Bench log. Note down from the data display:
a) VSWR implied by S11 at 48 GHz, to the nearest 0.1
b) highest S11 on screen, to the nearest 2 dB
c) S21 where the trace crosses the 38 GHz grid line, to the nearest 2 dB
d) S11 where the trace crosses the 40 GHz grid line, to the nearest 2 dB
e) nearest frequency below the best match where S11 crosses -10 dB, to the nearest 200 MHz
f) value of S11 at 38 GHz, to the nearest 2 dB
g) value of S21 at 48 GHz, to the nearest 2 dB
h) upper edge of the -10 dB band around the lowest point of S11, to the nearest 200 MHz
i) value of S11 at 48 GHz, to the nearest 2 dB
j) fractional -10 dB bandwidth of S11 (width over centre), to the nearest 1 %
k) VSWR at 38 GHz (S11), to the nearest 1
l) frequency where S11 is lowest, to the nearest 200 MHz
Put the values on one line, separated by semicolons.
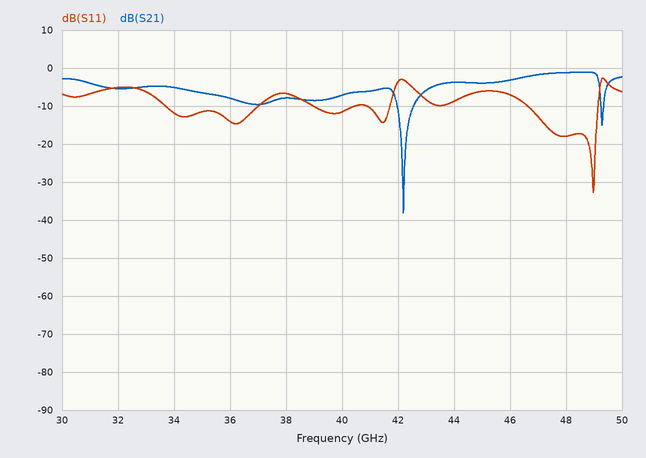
1.3; -2 dB; -8 dB; -12 dB; 46.6 GHz; -6 dB; -2 dB; 49.2 GHz; -18 dB; 5 %; 3; 49.0 GHz
